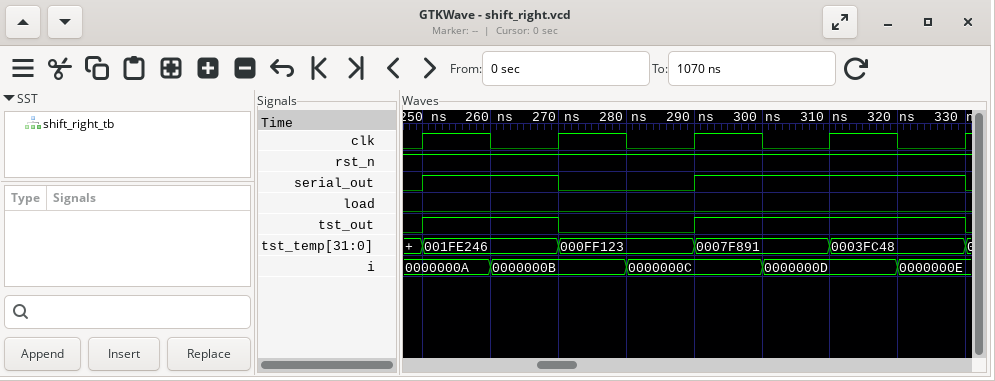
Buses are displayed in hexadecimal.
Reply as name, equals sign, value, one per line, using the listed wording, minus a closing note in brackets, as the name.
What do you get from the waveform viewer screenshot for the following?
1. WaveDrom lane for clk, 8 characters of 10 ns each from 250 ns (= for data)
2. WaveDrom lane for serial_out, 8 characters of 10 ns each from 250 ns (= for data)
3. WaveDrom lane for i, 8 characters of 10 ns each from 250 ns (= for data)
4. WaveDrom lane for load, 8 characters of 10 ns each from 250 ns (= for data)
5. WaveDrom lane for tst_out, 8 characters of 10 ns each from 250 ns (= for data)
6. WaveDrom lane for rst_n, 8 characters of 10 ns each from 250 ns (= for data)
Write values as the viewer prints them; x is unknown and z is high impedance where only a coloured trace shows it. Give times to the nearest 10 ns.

WaveDrom lane for clk, 8 characters of 10 ns each from 250 ns = {name: 'clk', wave: '10101010'}
WaveDrom lane for serial_out, 8 characters of 10 ns each from 250 ns = {name: 'serial_out', wave: '1.0.1...'}
WaveDrom lane for i, 8 characters of 10 ns each from 250 ns = {name: 'i', wave: '==.=.=.=', data: '0000000A 0000000B 0000000C 0000000D 0000000E'}
WaveDrom lane for load, 8 characters of 10 ns each from 250 ns = {name: 'load', wave: '0.......'}
WaveDrom lane for tst_out, 8 characters of 10 ns each from 250 ns = {name: 'tst_out', wave: '1.0.1...'}
WaveDrom lane for rst_n, 8 characters of 10 ns each from 250 ns = {name: 'rst_n', wave: '1.......'}
